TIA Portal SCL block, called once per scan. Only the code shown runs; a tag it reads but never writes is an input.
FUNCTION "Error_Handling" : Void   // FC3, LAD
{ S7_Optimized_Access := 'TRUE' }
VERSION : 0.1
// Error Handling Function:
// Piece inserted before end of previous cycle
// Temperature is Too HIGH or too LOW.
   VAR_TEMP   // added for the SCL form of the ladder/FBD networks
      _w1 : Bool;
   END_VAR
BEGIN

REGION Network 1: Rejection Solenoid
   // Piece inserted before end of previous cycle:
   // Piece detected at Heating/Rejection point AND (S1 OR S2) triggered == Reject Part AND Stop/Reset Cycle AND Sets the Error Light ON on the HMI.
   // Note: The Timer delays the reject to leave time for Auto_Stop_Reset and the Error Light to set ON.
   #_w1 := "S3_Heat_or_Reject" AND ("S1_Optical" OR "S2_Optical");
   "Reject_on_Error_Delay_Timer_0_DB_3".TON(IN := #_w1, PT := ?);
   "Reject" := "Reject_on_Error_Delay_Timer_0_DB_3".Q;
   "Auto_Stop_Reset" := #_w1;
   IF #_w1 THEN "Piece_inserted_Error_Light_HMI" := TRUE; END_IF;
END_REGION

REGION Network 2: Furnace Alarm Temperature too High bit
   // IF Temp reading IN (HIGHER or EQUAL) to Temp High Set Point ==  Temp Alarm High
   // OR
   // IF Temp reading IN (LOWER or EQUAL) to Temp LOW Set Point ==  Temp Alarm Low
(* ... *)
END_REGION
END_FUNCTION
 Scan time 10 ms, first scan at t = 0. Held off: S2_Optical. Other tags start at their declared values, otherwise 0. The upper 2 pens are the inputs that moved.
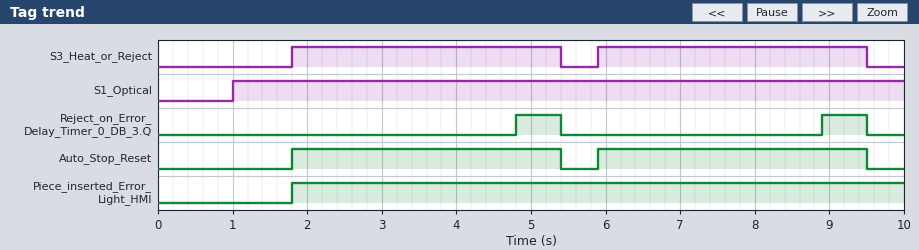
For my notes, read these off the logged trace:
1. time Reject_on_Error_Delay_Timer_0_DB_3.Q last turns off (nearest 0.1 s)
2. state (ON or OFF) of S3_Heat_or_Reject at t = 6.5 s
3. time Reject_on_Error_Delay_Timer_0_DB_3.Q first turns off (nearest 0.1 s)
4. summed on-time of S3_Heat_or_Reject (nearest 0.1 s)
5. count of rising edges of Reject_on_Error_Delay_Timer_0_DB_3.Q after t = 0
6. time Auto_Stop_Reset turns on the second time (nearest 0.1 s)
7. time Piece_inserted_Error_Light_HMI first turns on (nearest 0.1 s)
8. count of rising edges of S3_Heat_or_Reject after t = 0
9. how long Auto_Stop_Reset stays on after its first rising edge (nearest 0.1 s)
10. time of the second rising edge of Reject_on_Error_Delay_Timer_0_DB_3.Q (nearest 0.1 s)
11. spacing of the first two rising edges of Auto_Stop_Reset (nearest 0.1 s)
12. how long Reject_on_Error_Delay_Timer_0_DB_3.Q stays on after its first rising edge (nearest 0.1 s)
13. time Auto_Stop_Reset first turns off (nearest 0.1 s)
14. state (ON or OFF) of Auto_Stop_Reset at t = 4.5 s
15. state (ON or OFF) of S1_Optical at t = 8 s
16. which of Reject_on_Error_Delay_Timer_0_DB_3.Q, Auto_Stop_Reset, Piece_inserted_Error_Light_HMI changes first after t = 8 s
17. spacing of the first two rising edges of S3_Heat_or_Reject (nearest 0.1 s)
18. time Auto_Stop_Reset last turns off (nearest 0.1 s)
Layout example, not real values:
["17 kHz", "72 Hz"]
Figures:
["9.5 s", "ON", "5.4 s", "7.2 s", "2", "5.9 s", "1.8 s", "2", "3.6 s", "8.9 s", "4.1 s", "0.6 s", "5.4 s", "ON", "ON", "Reject_on_Error_Delay_Timer_0_DB_3.Q", "4.1 s", "9.5 s"]
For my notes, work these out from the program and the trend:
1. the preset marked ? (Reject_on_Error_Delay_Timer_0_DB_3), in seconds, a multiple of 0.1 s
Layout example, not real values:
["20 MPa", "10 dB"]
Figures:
["3.0 s"]
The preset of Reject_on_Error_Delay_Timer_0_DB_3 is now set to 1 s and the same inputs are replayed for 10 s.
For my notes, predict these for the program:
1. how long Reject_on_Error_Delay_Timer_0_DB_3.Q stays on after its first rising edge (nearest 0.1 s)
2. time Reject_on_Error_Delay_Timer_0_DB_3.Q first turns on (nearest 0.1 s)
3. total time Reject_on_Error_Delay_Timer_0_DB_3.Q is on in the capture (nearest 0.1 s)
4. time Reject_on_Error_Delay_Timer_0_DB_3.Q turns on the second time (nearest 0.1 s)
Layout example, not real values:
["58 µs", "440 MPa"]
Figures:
["2.6 s", "2.8 s", "5.2 s", "6.9 s"]
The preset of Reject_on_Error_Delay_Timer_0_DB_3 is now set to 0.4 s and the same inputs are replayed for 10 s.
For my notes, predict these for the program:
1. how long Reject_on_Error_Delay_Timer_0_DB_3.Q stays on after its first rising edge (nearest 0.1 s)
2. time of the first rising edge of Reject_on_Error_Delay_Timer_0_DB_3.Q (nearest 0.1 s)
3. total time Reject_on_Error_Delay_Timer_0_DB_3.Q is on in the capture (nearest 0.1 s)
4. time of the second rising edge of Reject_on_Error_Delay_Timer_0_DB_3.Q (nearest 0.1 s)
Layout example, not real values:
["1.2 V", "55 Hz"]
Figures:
["3.2 s", "2.2 s", "6.4 s", "6.3 s"]
